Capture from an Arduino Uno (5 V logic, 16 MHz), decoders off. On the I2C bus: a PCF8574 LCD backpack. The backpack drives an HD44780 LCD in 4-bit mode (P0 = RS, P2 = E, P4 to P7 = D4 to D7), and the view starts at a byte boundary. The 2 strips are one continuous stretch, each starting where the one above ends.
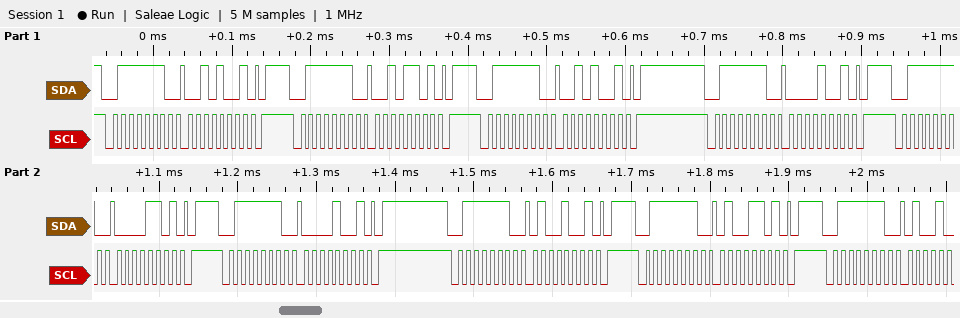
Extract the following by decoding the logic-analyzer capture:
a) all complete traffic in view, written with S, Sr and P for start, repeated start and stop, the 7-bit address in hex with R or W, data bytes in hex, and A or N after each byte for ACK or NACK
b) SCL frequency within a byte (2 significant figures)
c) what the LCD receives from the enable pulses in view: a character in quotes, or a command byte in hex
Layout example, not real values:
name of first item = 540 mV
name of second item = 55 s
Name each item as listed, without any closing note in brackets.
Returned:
all complete traffic in view, written with S, Sr and P for start, repeated start and stop, the 7-bit address in hex with R or W, data bytes in hex, and A or N after each byte for ACK or NACK = S 3FW A 29 A P S 3FW A 2D A P S 3FW A 29 A P S 3FW A 09 A P S 3FW A 0D A P S 3FW A 09 A P S 3FW A 49 A P S 3FW A 4D A P S 3FW A
SCL frequency within a byte = 100 kHz
what the LCD receives from the enable pulses in view: a character in quotes, or a command byte in hex = ' '
